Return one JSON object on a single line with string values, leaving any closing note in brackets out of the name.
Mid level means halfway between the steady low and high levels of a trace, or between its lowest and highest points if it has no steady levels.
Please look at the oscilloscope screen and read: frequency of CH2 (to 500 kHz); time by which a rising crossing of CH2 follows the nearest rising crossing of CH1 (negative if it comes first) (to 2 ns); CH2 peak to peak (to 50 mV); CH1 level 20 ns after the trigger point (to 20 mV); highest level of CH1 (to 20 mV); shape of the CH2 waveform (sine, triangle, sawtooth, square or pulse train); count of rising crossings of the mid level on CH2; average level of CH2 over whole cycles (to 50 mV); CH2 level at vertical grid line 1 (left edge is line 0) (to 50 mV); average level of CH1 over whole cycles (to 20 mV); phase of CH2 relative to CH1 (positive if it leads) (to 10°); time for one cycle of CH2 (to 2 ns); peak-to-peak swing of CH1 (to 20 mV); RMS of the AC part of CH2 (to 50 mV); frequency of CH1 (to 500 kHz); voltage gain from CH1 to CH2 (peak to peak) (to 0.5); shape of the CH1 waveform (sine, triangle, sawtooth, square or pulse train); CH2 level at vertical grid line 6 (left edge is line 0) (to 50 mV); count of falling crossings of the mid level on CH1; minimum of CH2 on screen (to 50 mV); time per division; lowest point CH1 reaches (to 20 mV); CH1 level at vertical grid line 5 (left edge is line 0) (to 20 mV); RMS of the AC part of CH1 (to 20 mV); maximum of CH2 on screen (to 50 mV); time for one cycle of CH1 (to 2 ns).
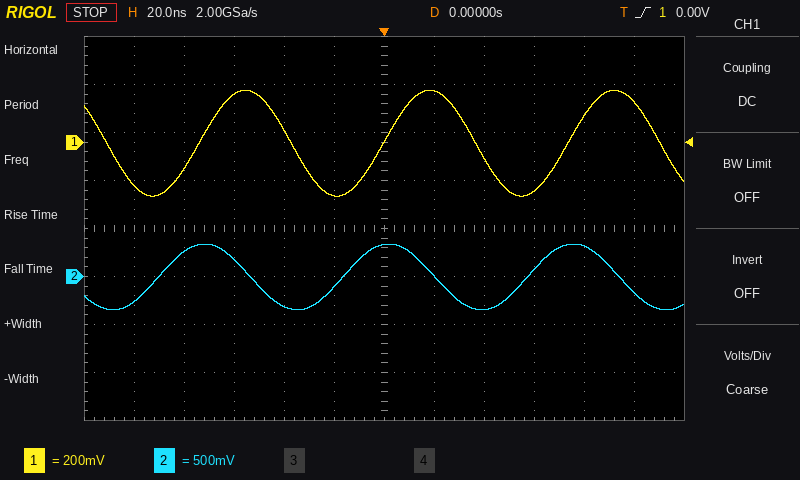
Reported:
{"frequency of CH2": "13.5 MHz", "time by which a rising crossing of CH2 follows the nearest rising crossing of CH1 (negative if it comes first)": "-16 ns", "CH2 peak to peak": "700 mV", "CH1 level 20 ns after the trigger point": "220 mV", "highest level of CH1": "220 mV", "shape of the CH2 waveform": "sine", "count of rising crossings of the mid level on CH2": "3", "average level of CH2 over whole cycles": "0 mV", "CH2 level at vertical grid line 1 (left edge is line 0)": "-250 mV", "average level of CH1 over whole cycles": "0 mV", "phase of CH2 relative to CH1 (positive if it leads)": "+80°", "time for one cycle of CH2": "74 ns", "peak-to-peak swing of CH1": "440 mV", "RMS of the AC part of CH2": "250 mV", "frequency of CH1": "13.5 MHz", "voltage gain from CH1 to CH2 (peak to peak)": "1.5", "shape of the CH1 waveform": "sine", "CH2 level at vertical grid line 6 (left edge is line 0)": "350 mV", "count of falling crossings of the mid level on CH1": "4", "minimum of CH2 on screen": "-350 mV", "time per division": "20 ns", "lowest point CH1 reaches": "-220 mV", "CH1 level at vertical grid line 5 (left edge is line 0)": "-220 mV", "RMS of the AC part of CH1": "160 mV", "maximum of CH2 on screen": "350 mV", "time for one cycle of CH1": "74 ns"}
